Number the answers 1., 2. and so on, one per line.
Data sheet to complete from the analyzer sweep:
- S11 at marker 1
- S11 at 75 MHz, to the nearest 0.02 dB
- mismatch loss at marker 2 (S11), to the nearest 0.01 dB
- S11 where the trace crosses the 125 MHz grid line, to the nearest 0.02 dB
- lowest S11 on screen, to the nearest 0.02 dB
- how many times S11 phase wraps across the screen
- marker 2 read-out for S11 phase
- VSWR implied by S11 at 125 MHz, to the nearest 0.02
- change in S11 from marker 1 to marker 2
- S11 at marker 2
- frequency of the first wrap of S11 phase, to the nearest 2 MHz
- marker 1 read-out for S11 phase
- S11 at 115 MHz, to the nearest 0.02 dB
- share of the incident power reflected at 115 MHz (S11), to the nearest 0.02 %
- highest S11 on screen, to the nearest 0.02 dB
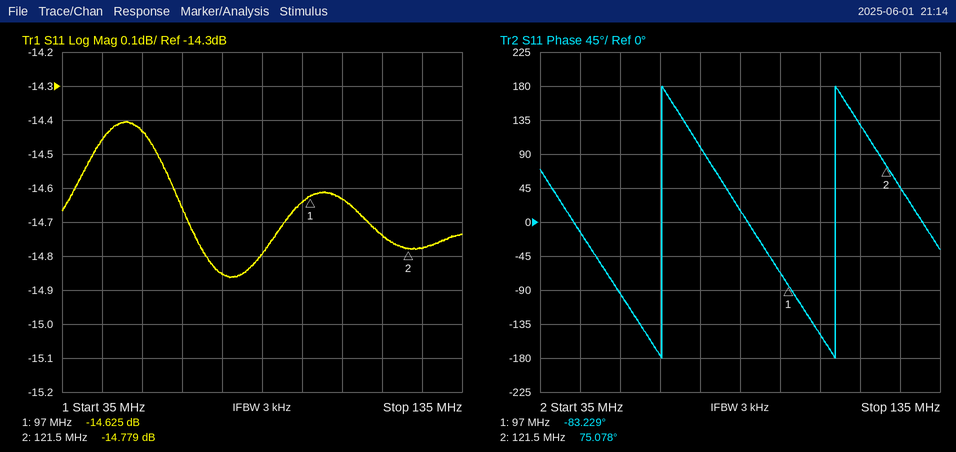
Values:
1. -14.625 dB
2. -14.86 dB
3. 0.15 dB
4. -14.78 dB
5. -14.86 dB
6. 2
7. 75.078°
8. 1.44
9. -0.154 dB
10. -14.779 dB
11. 66 MHz
12. -83.229°
13. -14.74 dB
14. 3.36 %
15. -14.40 dB
